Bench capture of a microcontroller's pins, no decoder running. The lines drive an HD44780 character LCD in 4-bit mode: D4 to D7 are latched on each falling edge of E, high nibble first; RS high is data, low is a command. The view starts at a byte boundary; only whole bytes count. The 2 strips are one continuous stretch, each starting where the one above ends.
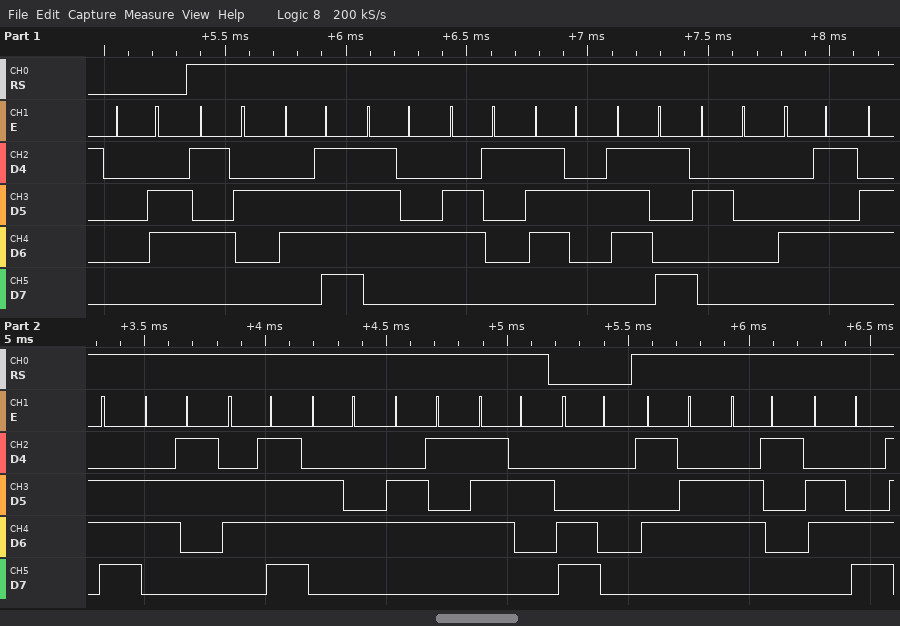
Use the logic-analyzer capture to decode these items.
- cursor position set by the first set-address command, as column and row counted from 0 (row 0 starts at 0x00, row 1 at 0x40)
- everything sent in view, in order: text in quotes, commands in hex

column 0, row 1
0x06 "Rotary Encoder" 0xC0 "Val"
